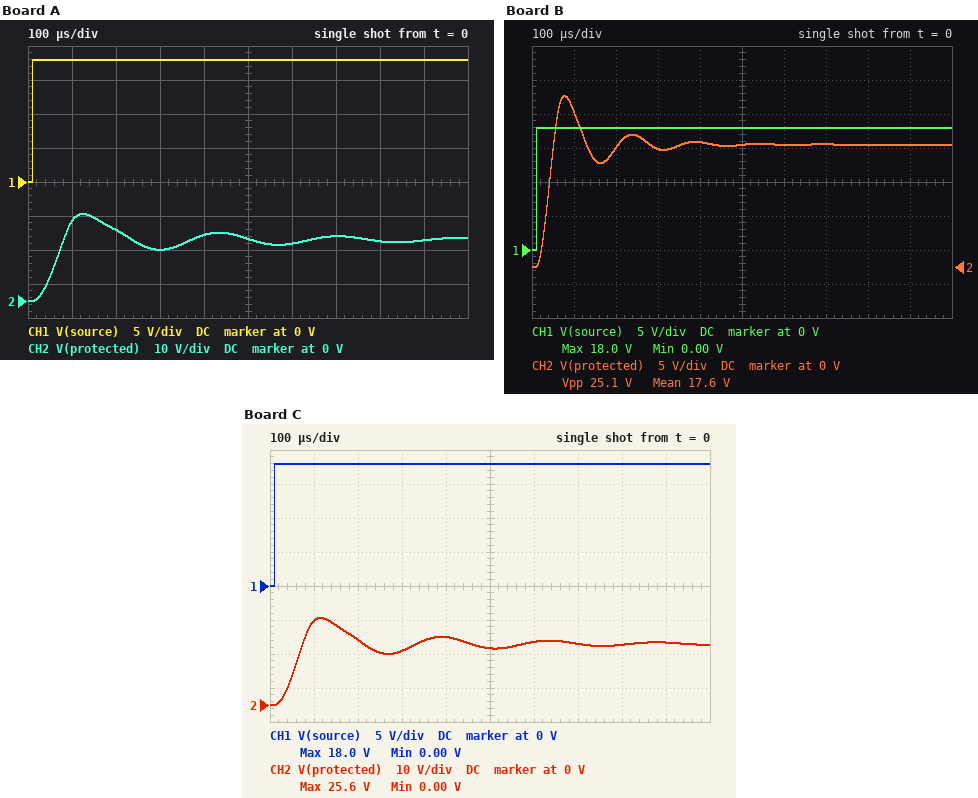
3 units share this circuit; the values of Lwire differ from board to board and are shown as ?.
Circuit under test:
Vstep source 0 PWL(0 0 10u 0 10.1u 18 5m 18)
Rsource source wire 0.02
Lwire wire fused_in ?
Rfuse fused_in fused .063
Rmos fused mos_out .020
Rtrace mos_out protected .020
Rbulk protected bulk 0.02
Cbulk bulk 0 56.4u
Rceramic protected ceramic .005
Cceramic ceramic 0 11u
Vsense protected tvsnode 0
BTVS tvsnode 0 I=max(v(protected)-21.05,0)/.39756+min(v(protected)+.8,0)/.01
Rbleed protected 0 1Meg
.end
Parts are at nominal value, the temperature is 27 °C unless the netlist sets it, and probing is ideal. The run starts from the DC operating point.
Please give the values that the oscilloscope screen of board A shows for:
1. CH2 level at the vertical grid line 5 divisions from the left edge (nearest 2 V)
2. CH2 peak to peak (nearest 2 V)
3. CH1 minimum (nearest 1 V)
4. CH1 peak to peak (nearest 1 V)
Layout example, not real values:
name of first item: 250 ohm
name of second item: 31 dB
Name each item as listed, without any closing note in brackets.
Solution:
CH2 level at the vertical grid line 5 divisions from the left edge: 18 V
CH2 peak to peak: 26 V
CH1 minimum: 0 V
CH1 peak to peak: 18 V
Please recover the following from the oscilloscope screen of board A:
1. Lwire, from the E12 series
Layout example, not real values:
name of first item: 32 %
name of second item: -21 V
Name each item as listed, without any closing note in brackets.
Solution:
Lwire, from the E12 series: 27 µH
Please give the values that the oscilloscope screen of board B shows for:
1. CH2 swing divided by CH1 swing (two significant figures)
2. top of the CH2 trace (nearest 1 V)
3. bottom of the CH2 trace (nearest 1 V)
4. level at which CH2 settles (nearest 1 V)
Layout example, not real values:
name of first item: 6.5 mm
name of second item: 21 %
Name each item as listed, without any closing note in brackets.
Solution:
CH2 swing divided by CH1 swing: 1.4
top of the CH2 trace: 25 V
bottom of the CH2 trace: 0 V
level at which CH2 settles: 18 V
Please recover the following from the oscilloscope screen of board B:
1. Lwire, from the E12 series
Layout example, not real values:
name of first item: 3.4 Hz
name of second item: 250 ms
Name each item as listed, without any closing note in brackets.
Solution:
Lwire, from the E12 series: 8.2 µH
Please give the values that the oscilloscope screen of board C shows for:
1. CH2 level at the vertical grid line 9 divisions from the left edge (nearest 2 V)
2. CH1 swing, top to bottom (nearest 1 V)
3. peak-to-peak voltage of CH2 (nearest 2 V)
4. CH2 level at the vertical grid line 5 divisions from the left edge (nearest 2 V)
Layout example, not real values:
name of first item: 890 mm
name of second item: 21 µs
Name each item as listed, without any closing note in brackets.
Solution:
CH2 level at the vertical grid line 9 divisions from the left edge: 18 V
CH1 swing, top to bottom: 18 V
peak-to-peak voltage of CH2: 26 V
CH2 level at the vertical grid line 5 divisions from the left edge: 16 V
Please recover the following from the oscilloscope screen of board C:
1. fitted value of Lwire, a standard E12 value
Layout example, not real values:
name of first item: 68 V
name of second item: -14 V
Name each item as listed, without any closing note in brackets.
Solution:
fitted value of Lwire, a standard E12 value: 22 µH
